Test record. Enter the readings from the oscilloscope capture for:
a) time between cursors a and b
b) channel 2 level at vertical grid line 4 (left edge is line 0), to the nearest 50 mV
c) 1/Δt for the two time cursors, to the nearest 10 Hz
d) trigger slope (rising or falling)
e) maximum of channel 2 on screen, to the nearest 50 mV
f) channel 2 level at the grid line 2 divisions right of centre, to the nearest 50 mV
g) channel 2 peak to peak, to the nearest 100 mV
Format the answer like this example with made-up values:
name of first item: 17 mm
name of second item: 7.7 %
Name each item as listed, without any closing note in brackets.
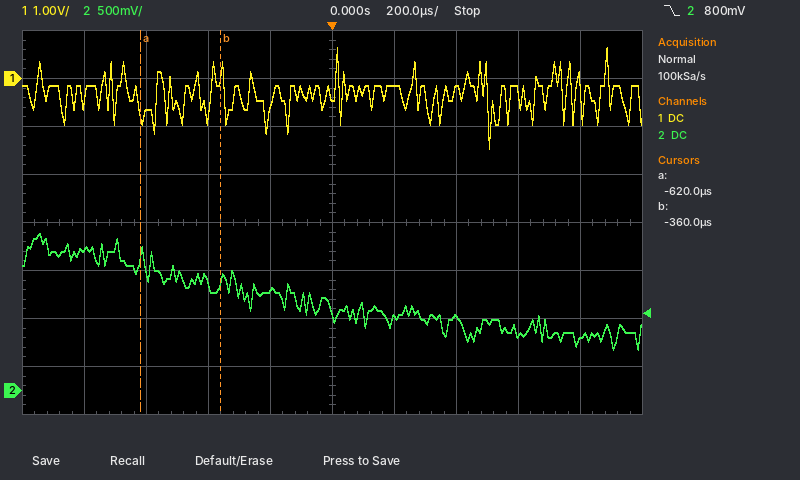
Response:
time between cursors a and b: 260 µs
channel 2 level at vertical grid line 4 (left edge is line 0), to the nearest 50 mV: 1.05 V
1/Δt for the two time cursors, to the nearest 10 Hz: 3.85 kHz
trigger slope: falling
maximum of channel 2 on screen, to the nearest 50 mV: 1.65 V
channel 2 level at the grid line 2 divisions right of centre, to the nearest 50 mV: 750 mV
channel 2 peak to peak, to the nearest 100 mV: 1.20 V
